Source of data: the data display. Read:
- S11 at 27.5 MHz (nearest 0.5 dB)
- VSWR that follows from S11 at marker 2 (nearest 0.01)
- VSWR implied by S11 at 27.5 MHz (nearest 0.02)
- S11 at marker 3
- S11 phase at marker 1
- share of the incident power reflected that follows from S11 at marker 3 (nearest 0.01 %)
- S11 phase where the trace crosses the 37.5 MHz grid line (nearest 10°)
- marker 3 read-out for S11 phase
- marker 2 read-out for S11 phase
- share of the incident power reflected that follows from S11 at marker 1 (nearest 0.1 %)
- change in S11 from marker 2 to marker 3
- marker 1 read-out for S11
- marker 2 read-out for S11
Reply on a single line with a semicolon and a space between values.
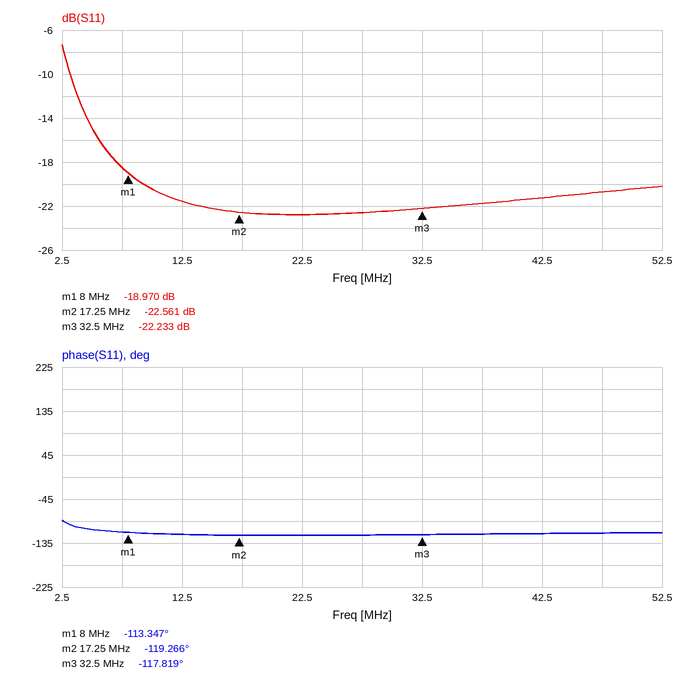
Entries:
-22.5 dB; 1.16; 1.16; -22.233 dB; -113.347°; 0.60 %; -120°; -117.819°; -119.266°; 1.3 %; 0.328 dB; -18.970 dB; -22.561 dB
